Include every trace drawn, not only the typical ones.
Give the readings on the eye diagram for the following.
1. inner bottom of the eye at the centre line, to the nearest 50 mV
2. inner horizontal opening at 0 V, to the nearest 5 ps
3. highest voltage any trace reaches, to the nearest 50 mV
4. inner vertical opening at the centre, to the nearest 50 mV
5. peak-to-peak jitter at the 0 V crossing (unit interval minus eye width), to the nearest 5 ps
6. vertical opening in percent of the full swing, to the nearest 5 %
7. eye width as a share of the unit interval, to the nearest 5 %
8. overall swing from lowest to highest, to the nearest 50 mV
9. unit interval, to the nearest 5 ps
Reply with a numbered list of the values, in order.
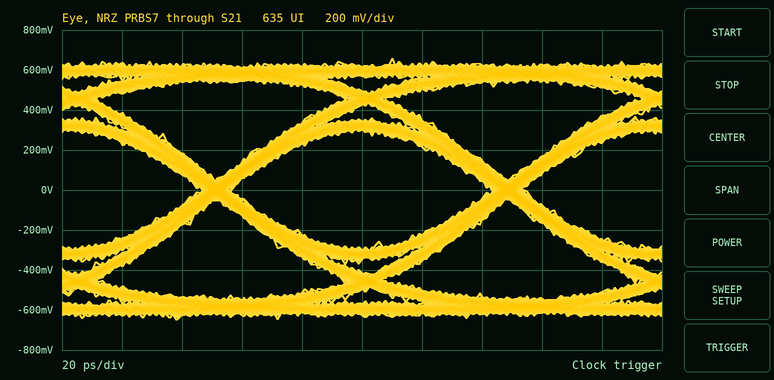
1. -300 mV
2. 85 ps
3. 650 mV
4. 600 mV
5. 10 ps
6. 45 %
7. 90 %
8. 1.30 V
9. 95 ps
